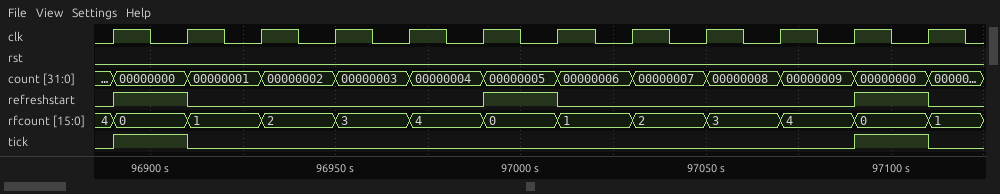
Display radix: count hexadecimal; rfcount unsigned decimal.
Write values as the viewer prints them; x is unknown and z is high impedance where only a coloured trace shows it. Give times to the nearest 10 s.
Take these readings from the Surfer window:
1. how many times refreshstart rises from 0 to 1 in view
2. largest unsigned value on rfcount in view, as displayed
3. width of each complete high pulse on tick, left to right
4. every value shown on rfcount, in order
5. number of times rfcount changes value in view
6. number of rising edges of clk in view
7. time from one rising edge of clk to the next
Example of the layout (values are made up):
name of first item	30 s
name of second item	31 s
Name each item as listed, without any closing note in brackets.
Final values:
how many times refreshstart rises from 0 to 1 in view	3
largest unsigned value on rfcount in view, as displayed	4
width of each complete high pulse on tick, left to right	20 s, 20 s
every value shown on rfcount, in order	4, 0, 1, 2, 3, 4, 0, 1, 2, 3, 4, 0, 1
number of times rfcount changes value in view	12
number of rising edges of clk in view	12
time from one rising edge of clk to the next	20 s
